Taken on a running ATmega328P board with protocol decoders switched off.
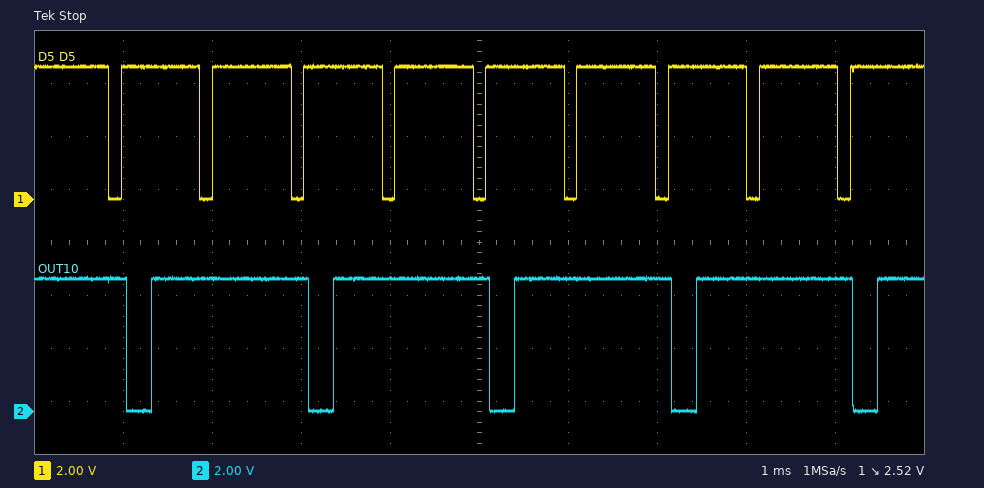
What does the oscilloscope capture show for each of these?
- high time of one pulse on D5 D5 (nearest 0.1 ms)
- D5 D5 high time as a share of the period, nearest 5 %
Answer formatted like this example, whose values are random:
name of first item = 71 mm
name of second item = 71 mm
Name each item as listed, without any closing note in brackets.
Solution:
high time of one pulse on D5 D5 = 0.9 ms
D5 D5 high time as a share of the period, nearest 5 % = 85 %
